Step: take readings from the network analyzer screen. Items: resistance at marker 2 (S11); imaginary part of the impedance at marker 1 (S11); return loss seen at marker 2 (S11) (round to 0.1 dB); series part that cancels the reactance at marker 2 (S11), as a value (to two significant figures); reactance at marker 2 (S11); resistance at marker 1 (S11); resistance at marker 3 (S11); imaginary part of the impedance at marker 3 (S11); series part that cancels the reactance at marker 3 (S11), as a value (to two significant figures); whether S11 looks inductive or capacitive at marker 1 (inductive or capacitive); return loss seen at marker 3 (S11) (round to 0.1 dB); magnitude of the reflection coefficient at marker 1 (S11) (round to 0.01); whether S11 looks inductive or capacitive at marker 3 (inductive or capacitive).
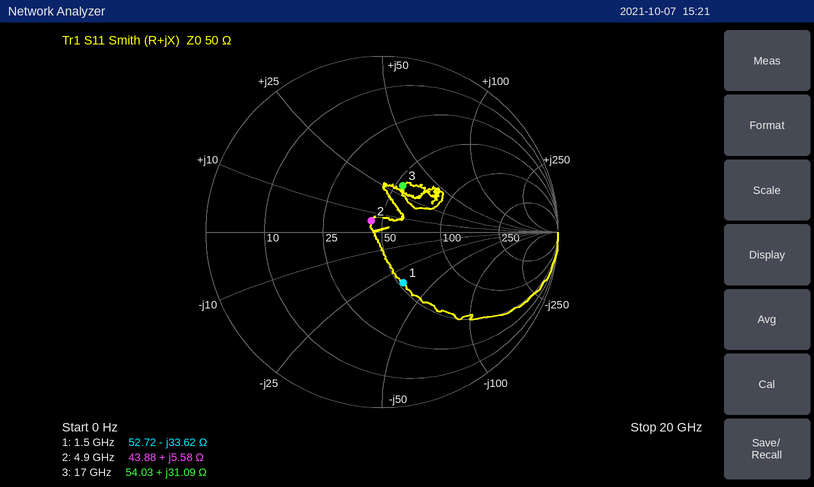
43.88 Ω
-33.62 Ω
21.1 dB
5.8 pF
+5.58 Ω
52.72 Ω
54.03 Ω
+31.09 Ω
300 fF
capacitive
10.8 dB
0.31
inductive
